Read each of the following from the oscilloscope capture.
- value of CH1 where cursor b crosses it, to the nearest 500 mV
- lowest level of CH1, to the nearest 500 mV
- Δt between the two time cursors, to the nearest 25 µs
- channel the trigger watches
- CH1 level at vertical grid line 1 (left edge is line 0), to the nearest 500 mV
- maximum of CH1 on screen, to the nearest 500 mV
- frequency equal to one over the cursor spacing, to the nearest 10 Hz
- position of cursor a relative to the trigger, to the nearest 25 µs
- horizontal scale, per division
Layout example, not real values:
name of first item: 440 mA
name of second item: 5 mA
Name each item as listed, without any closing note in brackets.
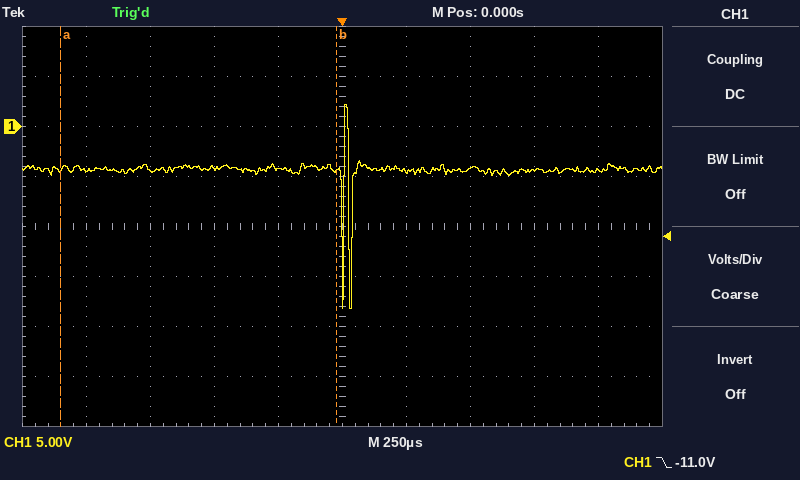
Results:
value of CH1 where cursor b crosses it, to the nearest 500 mV: -4.5 V
lowest level of CH1, to the nearest 500 mV: -18.0 V
Δt between the two time cursors, to the nearest 25 µs: 1.075 ms
channel the trigger watches: CH1
CH1 level at vertical grid line 1 (left edge is line 0), to the nearest 500 mV: -4.5 V
maximum of CH1 on screen, to the nearest 500 mV: 2.0 V
frequency equal to one over the cursor spacing, to the nearest 10 Hz: 930 Hz
position of cursor a relative to the trigger, to the nearest 25 µs: -1.100 ms
horizontal scale, per division: 250 µs
